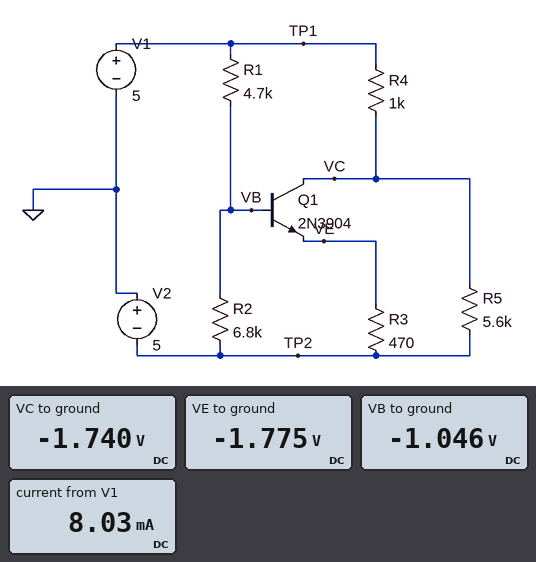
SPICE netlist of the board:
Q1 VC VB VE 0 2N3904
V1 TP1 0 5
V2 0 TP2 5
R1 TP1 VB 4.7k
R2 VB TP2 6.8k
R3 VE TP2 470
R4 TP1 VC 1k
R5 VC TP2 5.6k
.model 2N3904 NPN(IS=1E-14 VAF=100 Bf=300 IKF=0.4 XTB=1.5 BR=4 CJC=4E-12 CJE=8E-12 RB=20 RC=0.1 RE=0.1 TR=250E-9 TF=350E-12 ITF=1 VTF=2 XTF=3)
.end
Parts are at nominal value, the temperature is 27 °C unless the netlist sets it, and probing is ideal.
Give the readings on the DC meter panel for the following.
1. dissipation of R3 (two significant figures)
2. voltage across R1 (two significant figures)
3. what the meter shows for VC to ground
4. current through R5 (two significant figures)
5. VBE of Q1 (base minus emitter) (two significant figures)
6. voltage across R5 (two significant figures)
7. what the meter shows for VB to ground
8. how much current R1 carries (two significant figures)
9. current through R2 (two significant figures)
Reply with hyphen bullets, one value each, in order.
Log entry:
- 22 mW
- 6.0 V
- -1.740 V
- 580 µA
- 730 mV
- 3.3 V
- -1.046 V
- 1.3 mA
- 580 µA
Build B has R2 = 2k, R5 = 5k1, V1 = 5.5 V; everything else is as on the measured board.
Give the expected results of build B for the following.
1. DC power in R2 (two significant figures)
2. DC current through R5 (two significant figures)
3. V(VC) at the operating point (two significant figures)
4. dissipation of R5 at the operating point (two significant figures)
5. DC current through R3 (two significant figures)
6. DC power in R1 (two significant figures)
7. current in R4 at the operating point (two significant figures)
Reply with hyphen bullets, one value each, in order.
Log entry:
- 4.8 mW
- 880 µA
- -500 mV
- 4.0 mW
- 5.1 mA
- 12 mW
- 6.0 mA
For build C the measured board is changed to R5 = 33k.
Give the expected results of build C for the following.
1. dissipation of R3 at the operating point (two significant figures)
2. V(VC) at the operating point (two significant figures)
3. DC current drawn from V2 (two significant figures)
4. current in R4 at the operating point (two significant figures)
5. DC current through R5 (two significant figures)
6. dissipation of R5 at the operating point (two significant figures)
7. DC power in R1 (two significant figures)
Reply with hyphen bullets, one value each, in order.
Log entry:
- 24 mW
- -1.6 V
- 7.9 mA
- 6.6 mA
- 100 µA
- 350 µW
- 7.4 mW
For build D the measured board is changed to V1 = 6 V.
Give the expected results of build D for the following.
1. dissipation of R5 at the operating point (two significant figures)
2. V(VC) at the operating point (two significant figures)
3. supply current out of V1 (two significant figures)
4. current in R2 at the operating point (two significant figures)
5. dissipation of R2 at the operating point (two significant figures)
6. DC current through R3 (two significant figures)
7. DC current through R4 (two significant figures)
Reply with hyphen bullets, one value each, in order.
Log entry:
- 2.3 mW
- -1.4 V
- 8.8 mA
- 630 µA
- 2.7 mW
- 7.6 mA
- 7.4 mA
